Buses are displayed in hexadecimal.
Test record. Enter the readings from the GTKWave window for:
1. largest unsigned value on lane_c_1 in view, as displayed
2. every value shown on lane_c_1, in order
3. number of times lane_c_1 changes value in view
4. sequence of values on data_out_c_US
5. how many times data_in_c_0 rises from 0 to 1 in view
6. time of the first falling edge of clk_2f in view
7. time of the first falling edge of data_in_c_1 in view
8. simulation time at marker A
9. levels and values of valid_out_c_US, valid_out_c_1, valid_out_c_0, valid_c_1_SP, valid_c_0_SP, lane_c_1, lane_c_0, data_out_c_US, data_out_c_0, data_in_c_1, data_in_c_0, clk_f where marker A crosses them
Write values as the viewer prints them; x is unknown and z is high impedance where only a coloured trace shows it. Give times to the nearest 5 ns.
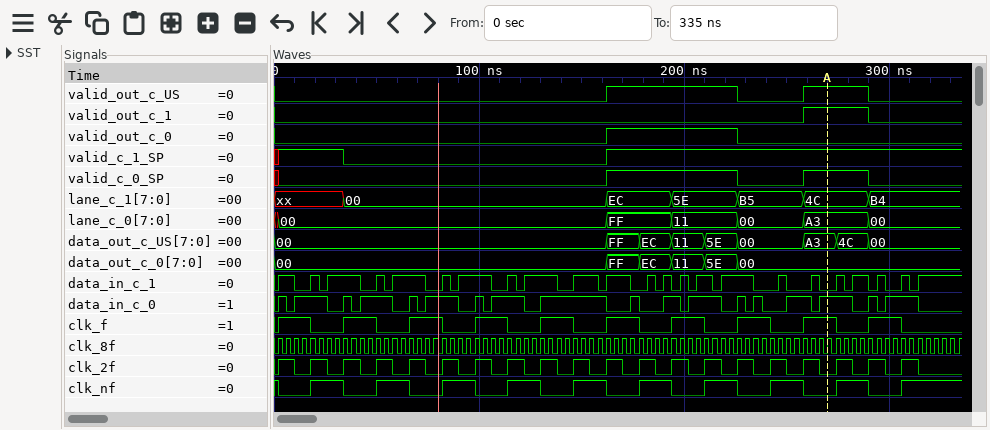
EC
xx, 00, EC, 5E, B5, 4C, B4
6
00, FF, EC, 11, 5E, 00, A3, 4C, 00
18
10 ns
10 ns
270 ns
valid_out_c_US=1, valid_out_c_1=1, valid_out_c_0=0, valid_c_1_SP=1, valid_c_0_SP=1, lane_c_1=4C, lane_c_0=A3, data_out_c_US=A3, data_out_c_0=00, data_in_c_1=0, data_in_c_0=1, clk_f=1
